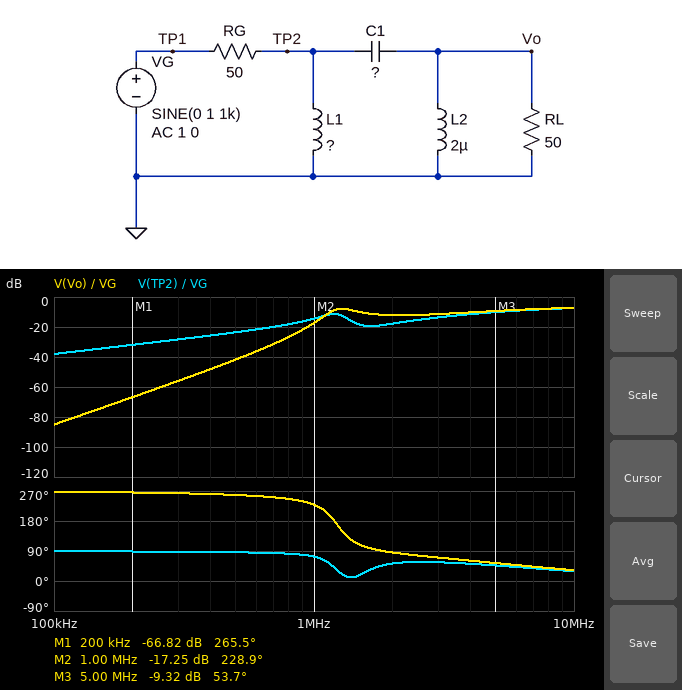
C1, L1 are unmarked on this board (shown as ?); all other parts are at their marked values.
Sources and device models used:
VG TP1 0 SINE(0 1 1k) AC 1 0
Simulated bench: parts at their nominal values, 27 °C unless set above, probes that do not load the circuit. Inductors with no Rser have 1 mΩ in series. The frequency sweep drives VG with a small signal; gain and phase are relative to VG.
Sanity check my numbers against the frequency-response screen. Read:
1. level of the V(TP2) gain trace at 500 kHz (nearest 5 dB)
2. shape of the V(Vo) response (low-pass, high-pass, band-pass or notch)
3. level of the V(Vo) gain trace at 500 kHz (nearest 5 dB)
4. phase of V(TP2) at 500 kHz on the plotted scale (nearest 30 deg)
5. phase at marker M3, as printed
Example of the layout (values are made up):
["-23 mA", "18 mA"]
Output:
["-25 dB", "high-pass", "-40 dB", "90 deg", "53.7 deg"]
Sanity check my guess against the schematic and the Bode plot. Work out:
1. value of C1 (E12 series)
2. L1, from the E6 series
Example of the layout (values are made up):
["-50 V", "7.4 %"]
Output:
["5.6 nF", "1 µH"]
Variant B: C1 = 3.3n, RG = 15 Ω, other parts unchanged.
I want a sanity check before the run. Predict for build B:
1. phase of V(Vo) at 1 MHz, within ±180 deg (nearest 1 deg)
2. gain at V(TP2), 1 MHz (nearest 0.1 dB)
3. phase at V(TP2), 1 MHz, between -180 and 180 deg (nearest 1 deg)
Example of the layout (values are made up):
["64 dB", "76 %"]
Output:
["-136 deg", "-7.0 dB", "62 deg"]
